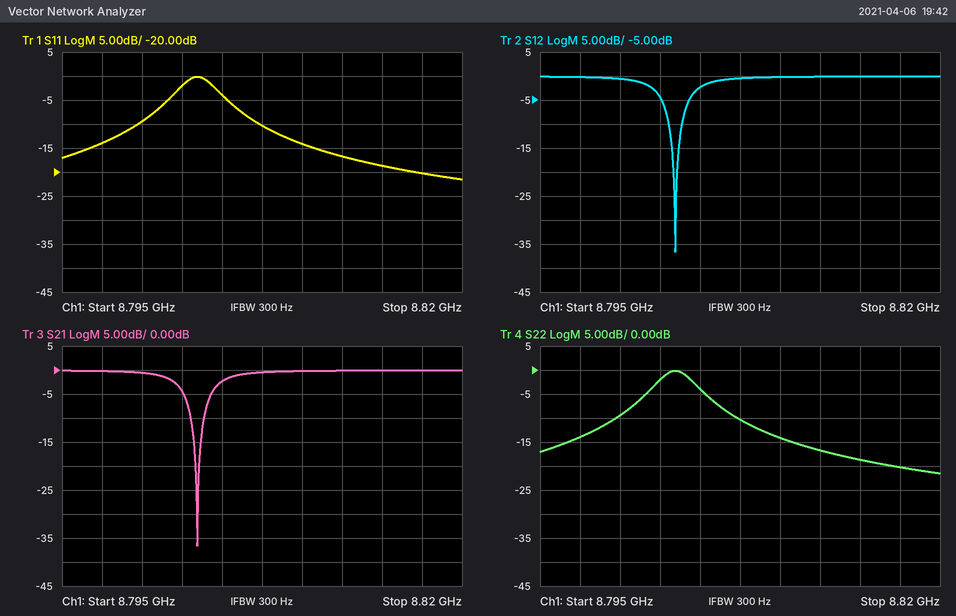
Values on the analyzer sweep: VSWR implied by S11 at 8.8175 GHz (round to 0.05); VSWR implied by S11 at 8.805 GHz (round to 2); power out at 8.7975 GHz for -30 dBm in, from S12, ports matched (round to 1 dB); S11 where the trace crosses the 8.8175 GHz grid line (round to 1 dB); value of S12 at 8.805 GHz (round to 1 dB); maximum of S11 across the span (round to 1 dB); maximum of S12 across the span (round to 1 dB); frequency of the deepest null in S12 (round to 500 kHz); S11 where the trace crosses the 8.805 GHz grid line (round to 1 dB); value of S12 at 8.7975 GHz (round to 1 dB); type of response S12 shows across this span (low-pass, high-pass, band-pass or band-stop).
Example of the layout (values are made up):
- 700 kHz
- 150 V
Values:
- 1.20
- 4
- -30 dBm
- -20 dB
- -2 dB
- 0 dB
- 0 dB
- 8.8035 GHz
- -4 dB
- 0 dB
- band-stop
